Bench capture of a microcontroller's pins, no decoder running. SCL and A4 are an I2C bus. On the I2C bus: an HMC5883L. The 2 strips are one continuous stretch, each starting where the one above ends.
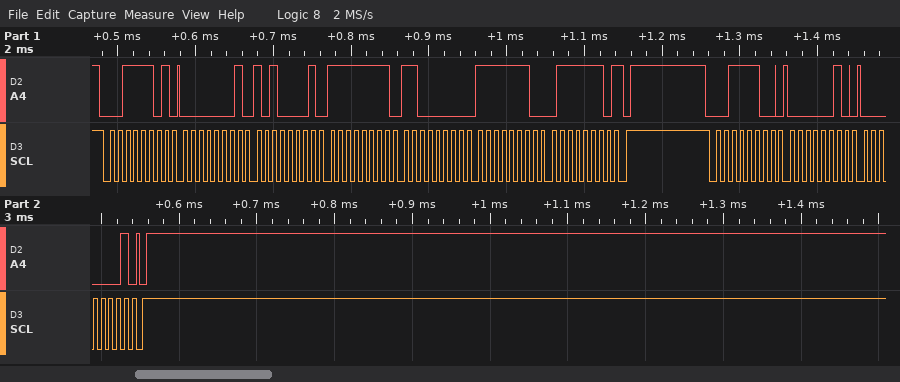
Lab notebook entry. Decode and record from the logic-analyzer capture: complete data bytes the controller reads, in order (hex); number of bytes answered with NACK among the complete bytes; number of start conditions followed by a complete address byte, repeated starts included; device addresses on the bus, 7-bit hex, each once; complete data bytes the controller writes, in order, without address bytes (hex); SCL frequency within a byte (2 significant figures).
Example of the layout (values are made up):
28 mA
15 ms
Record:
01 A1 FF C0 FE 7E
1
2
0x1E
02 01
100 kHz
